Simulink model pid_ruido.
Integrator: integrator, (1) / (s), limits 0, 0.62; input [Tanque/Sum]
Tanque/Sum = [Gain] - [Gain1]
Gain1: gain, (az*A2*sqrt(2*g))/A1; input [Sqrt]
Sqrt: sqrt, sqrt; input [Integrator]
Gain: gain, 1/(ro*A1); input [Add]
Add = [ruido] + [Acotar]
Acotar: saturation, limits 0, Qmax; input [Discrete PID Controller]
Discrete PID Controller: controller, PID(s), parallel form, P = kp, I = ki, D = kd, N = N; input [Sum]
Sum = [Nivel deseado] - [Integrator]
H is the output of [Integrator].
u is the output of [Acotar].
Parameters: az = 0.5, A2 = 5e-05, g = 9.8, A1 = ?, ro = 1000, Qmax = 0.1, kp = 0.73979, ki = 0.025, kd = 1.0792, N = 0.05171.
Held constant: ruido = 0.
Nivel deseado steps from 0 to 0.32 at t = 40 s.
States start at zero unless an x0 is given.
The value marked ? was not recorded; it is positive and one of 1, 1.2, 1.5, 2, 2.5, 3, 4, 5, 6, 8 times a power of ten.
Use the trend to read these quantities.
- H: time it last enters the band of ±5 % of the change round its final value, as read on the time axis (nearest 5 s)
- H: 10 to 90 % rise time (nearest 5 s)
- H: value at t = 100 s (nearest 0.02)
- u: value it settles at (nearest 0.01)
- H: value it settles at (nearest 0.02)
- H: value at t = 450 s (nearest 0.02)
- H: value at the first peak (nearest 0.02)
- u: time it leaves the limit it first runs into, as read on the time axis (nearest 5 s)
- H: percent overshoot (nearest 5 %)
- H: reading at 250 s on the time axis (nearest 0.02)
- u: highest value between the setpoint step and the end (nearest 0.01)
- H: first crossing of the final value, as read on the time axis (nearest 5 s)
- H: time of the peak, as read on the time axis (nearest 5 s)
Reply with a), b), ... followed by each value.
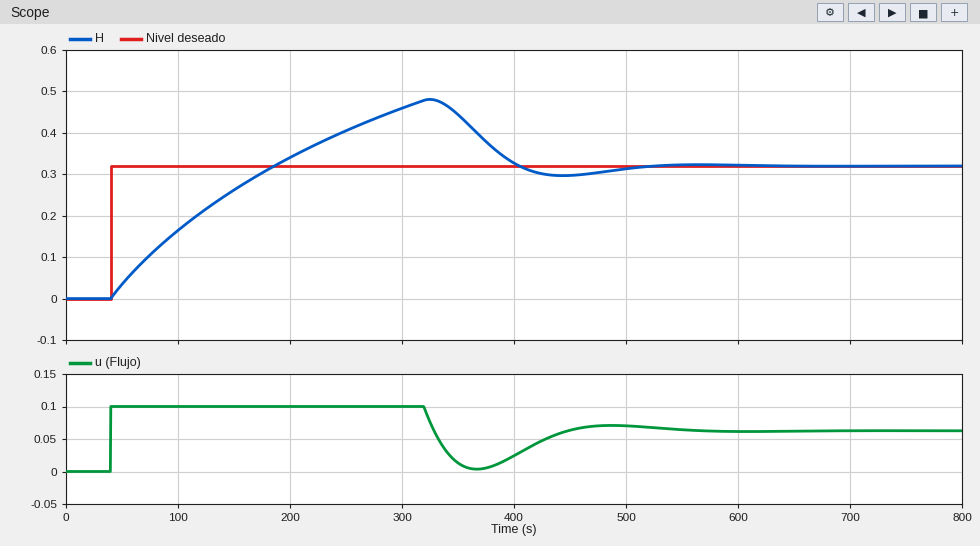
a) 475 s
b) 115 s
c) 0.16
d) 0.06
e) 0.32
f) 0.30
g) 0.48
h) 320 s
i) 50 %
j) 0.40
k) 0.10
l) 185 s
m) 325 s
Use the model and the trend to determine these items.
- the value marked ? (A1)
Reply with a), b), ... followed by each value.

a) 0.025
